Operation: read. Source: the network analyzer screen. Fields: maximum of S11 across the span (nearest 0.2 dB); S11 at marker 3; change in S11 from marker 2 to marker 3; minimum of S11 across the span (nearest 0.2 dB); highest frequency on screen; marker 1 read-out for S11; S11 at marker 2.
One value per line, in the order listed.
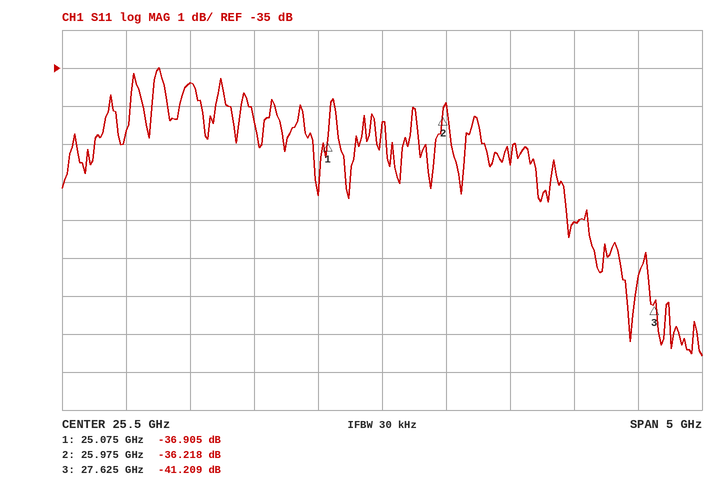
-35.0 dB
-41.209 dB
-4.991 dB
-42.6 dB
28 GHz
-36.905 dB
-36.218 dB
